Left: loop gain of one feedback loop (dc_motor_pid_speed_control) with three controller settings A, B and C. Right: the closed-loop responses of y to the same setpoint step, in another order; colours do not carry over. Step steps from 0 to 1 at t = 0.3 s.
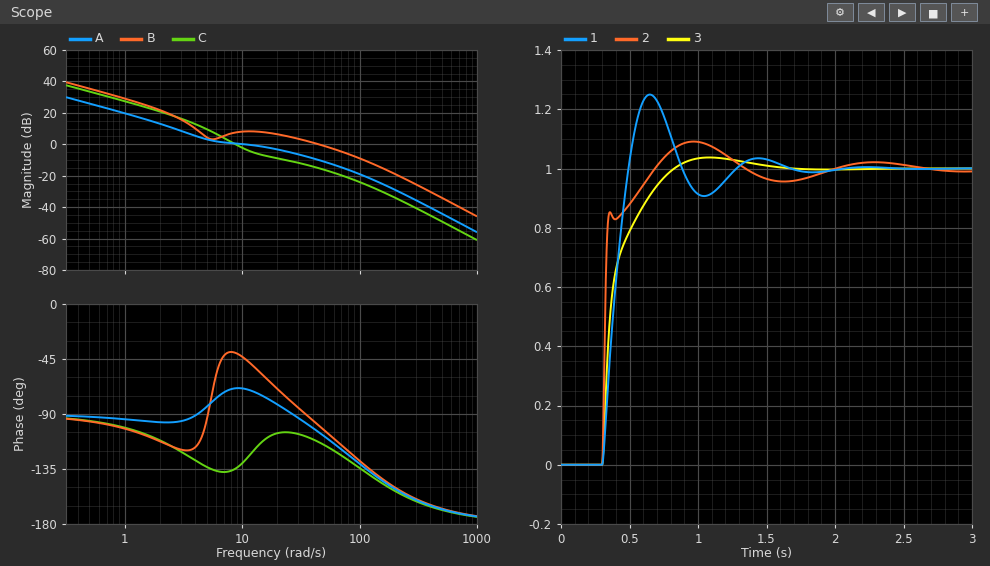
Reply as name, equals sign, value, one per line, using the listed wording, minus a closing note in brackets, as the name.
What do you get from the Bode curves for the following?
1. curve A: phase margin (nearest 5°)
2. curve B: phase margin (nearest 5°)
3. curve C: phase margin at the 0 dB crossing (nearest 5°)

curve A: phase margin = 110°
curve B: phase margin = 80°
curve C: phase margin at the 0 dB crossing = 45°
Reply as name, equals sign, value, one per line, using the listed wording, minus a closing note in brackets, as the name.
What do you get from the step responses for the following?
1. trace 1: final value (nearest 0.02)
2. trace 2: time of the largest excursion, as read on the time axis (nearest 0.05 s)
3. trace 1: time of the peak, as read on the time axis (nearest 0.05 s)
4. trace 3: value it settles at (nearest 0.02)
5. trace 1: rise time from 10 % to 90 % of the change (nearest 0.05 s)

trace 1: final value = 1.00
trace 2: time of the largest excursion, as read on the time axis = 0.95 s
trace 1: time of the peak, as read on the time axis = 0.65 s
trace 3: value it settles at = 1.00
trace 1: rise time from 10 % to 90 % of the change = 0.15 s
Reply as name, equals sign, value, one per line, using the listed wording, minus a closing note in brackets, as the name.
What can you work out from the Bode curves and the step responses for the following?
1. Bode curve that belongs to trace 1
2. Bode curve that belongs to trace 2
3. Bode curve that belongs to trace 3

Bode curve that belongs to trace 1 = C
Bode curve that belongs to trace 2 = B
Bode curve that belongs to trace 3 = A
